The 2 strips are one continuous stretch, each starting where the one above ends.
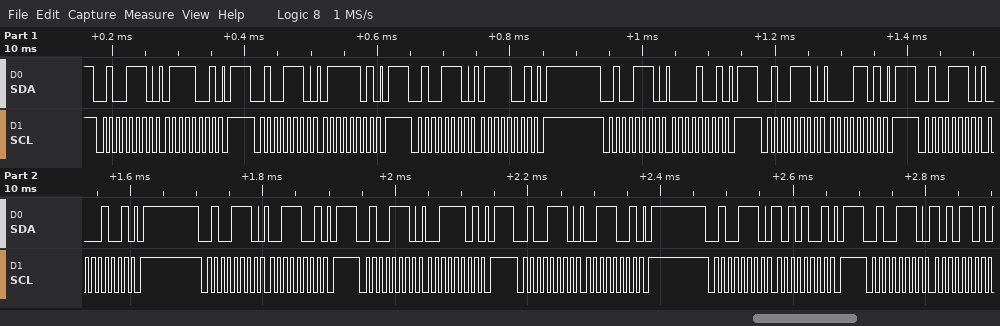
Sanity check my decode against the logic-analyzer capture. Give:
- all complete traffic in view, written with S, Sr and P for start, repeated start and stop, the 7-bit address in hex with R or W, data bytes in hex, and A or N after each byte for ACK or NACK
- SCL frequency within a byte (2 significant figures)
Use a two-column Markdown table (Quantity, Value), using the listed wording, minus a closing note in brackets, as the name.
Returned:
| Quantity | Value |
|---|---|
| all complete traffic in view, written with S, Sr and P for start, repeated start and stop, the 7-bit address in hex with R or W, data bytes in hex, and A or N after each byte for ACK or NACK | S 27W A 79 A P S 27W A 7D A P S 27W A 79 A P S 27W A 09 A P S 27W A 0D A P S 27W A 09 A P S 27W A 39 A P S 27W A 3D A P S 27W A 39 A P S 27W A A9 A P S 27W A AD A |
| SCL frequency within a byte | 100 kHz |
